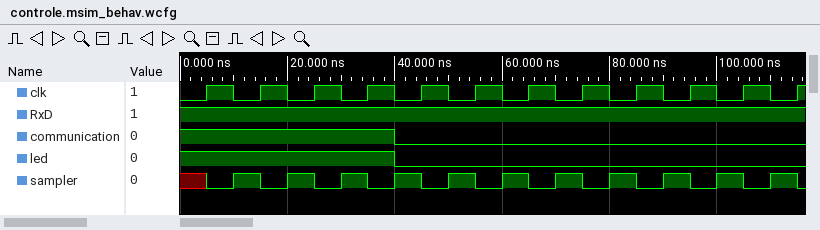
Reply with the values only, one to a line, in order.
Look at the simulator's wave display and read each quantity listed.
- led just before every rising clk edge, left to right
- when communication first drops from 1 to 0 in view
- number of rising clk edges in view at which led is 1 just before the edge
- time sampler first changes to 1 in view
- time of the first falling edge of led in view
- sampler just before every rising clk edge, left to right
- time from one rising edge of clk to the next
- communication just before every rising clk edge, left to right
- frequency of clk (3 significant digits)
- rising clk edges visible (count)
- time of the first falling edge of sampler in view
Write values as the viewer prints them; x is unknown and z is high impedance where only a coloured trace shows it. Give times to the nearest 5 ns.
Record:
1 1 1 1 0 0 0 0 0 0 0 0
40 ns
4
10 ns
40 ns
x 1 1 1 1 1 1 1 1 1 1 1
10 ns
1 1 1 1 0 0 0 0 0 0 0 0
100 MHz
12
15 ns
